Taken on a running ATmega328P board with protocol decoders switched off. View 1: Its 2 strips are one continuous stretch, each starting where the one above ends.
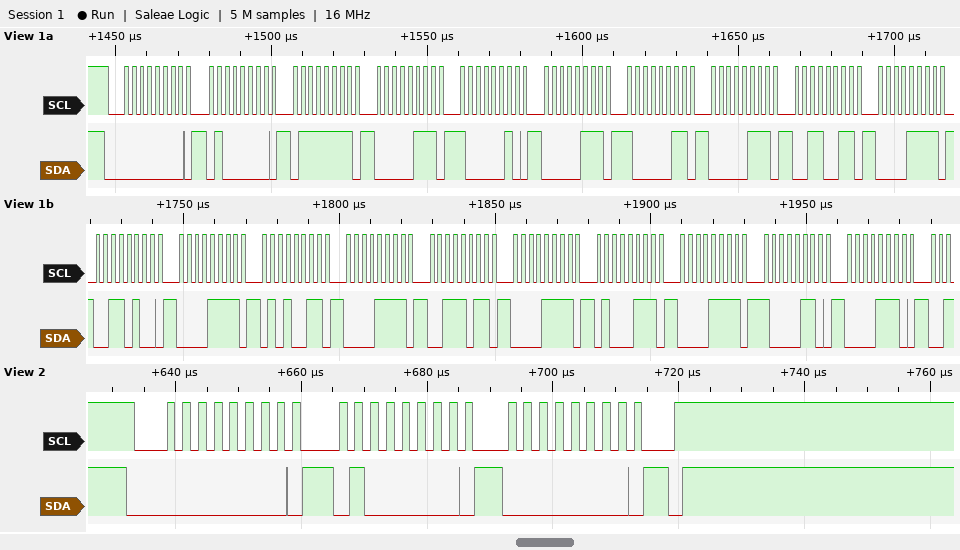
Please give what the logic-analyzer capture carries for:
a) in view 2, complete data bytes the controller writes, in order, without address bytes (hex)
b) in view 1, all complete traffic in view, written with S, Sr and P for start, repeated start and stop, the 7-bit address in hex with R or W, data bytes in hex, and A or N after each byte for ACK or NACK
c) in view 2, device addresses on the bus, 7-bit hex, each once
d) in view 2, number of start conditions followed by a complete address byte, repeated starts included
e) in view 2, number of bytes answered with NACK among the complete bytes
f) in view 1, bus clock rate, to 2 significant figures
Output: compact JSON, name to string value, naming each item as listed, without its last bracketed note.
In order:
{"in view 2, complete data bytes the controller writes, in order, without address bytes": "40 00", "in view 1, all complete traffic in view, written with S, Sr and P for start, repeated start and stop, the 7-bit address in hex with R or W, data bytes in hex, and A or N after each byte for ACK or NACK": "S 00W A 40 A 7F A 07 A 82 A 07 A 83 A 07 A 33 A 0F A 34 A 0F A 53 A 0F A 3B A 0F A 47 A 0F A 86 A 0E A", "in view 2, device addresses on the bus, 7-bit hex, each once": "0x00", "in view 2, number of start conditions followed by a complete address byte, repeated starts included": "1", "in view 2, number of bytes answered with NACK among the complete bytes": "0", "in view 1, bus clock rate, to 2 significant figures": "400 kHz"}
